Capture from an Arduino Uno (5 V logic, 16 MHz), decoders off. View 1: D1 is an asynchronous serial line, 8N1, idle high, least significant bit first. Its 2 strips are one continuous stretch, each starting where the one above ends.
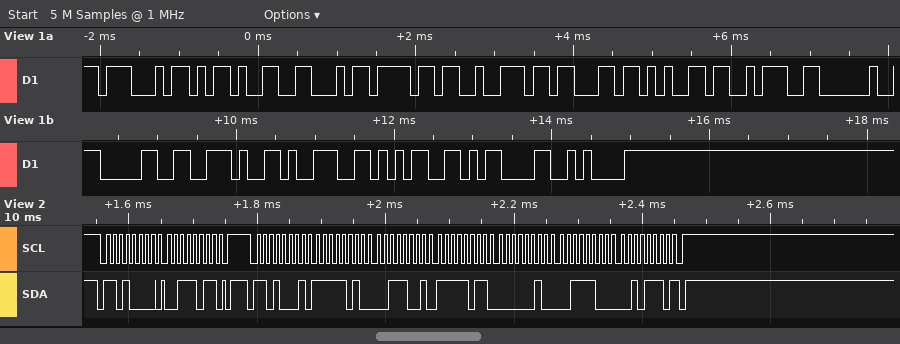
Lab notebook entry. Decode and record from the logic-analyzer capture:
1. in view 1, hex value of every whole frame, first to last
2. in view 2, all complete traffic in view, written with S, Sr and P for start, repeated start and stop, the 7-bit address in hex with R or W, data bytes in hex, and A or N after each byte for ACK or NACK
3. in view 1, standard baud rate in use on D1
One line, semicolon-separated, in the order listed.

0x47 0x2D 0x46 0x6F 0x72 0x63 0x65 0x3A 0x20 0x30 0x2E 0x39 0x35 0x0D 0x0A; S 68W A 3B A P S 68R A FA A 39 A FB A 02 A 3C A 2E N P; 9600 baud
